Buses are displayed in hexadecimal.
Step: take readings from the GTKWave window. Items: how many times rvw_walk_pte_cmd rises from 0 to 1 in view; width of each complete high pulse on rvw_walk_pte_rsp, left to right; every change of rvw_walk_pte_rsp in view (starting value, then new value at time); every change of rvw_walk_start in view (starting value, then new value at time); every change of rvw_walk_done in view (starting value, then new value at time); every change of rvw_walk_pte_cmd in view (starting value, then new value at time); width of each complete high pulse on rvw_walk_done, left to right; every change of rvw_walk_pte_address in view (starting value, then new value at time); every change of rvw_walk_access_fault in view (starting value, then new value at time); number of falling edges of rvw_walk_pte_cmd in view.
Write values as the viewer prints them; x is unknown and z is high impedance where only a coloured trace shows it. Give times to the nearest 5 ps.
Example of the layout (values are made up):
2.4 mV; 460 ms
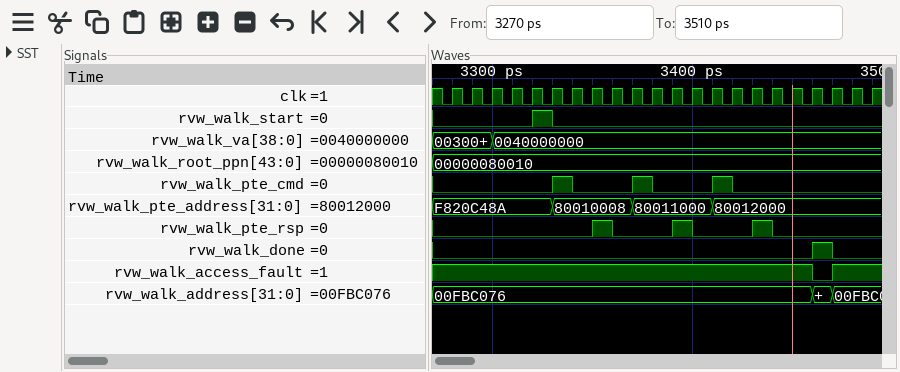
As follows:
3; 10 ps, 10 ps, 10 ps; 0, 1 at 3350 ps, 0 at 3360 ps, 1 at 3390 ps, 0 at 3400 ps, 1 at 3430 ps, 0 at 3440 ps; 0, 1 at 3320 ps, 0 at 3330 ps; 0, 1 at 3460 ps, 0 at 3470 ps; 0, 1 at 3330 ps, 0 at 3340 ps, 1 at 3370 ps, 0 at 3380 ps, 1 at 3410 ps, 0 at 3420 ps; 10 ps; F820C48A, 80010008 at 3330 ps, 80011000 at 3370 ps, 80012000 at 3410 ps; 1, 0 at 3460 ps, 1 at 3470 ps; 3
